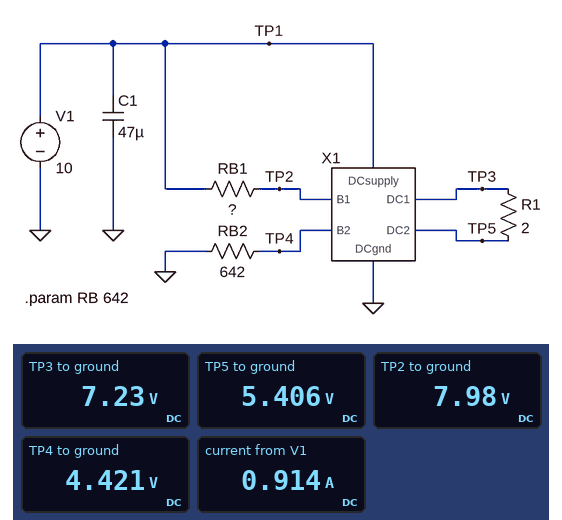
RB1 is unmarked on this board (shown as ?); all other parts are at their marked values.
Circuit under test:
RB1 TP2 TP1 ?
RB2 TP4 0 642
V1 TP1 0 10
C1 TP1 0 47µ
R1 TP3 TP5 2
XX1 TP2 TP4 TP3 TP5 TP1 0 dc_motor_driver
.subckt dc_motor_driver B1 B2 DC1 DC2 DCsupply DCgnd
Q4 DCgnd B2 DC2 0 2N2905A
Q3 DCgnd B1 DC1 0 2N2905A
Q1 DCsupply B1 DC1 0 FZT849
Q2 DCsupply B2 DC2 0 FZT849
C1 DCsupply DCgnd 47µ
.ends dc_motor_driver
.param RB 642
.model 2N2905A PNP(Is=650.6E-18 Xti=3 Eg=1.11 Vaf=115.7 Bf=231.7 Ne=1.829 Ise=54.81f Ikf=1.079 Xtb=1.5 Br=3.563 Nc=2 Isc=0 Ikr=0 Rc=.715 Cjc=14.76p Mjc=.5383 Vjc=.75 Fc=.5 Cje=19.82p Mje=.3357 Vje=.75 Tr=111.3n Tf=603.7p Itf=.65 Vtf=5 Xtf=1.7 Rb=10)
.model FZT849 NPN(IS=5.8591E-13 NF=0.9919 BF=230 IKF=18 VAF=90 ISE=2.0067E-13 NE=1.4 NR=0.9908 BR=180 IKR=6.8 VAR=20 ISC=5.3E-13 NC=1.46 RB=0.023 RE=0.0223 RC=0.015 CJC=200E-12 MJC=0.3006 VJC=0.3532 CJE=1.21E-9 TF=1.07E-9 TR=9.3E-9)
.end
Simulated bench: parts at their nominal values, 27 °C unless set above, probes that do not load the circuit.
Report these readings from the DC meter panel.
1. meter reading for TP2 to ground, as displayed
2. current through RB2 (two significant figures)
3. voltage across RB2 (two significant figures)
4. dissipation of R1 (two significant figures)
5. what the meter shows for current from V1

7.98 V
6.9 mA
4.4 V
1.7 W
0.914 A
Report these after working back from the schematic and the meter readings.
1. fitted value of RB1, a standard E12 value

470 Ω
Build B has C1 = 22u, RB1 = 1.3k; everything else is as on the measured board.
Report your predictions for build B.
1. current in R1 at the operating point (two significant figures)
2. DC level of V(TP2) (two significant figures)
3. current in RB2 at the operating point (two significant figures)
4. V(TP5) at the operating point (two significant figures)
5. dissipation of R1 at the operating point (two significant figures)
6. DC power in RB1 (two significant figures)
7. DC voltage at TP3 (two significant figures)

680 mA
6.0 V
4.6 mA
3.9 V
920 mW
12 mW
5.3 V
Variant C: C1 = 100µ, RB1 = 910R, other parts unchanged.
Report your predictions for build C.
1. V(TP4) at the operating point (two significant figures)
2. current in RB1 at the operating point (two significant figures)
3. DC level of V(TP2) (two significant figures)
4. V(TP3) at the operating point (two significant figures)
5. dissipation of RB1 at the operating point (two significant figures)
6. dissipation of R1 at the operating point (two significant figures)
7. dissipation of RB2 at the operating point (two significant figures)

3.5 V
3.6 mA
6.8 V
6.0 V
12 mW
1.2 W
19 mW
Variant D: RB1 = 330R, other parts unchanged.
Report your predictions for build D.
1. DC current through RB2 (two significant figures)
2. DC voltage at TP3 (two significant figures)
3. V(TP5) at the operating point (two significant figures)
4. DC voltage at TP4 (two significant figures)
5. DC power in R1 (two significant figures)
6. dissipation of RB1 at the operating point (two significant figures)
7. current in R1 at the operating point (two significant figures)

7.5 mA
7.7 V
5.8 V
4.8 V
1.9 W
7.0 mW
970 mA
